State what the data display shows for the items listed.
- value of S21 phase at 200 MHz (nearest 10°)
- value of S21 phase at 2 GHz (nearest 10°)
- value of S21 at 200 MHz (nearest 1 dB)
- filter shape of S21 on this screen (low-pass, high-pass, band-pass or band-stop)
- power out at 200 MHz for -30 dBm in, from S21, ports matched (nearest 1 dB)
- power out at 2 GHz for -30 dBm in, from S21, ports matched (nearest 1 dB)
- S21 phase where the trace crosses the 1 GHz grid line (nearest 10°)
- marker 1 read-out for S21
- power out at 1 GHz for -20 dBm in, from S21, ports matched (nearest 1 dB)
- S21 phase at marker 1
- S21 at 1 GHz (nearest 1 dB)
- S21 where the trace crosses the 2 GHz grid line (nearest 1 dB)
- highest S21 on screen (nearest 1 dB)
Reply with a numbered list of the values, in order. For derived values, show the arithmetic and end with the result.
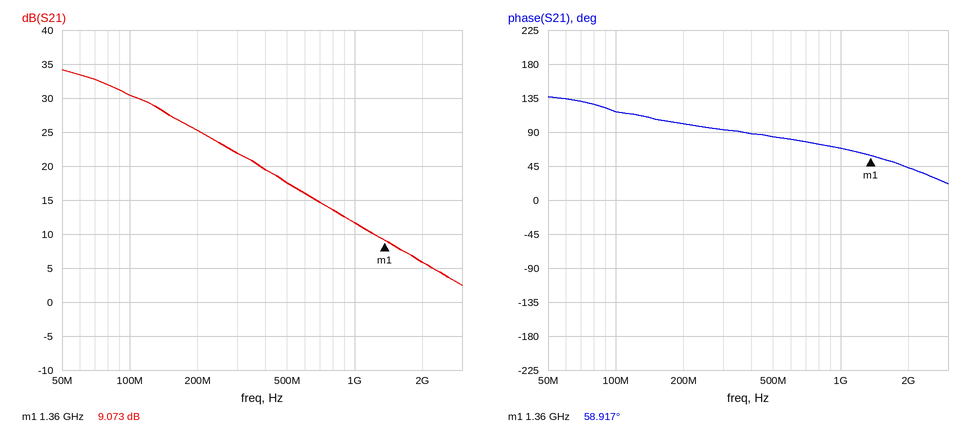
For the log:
1. 100°
2. 40°
3. 25 dB
4. low-pass
5. -30 dBm + (25 dB) = -5 dBm
6. -30 dBm + (6 dB) = -24 dBm
7. 70°
8. 9.073 dB
9. -20 dBm + (12 dB) = -8 dBm
10. 58.917°
11. 12 dB
12. 6 dB
13. 34 dB
